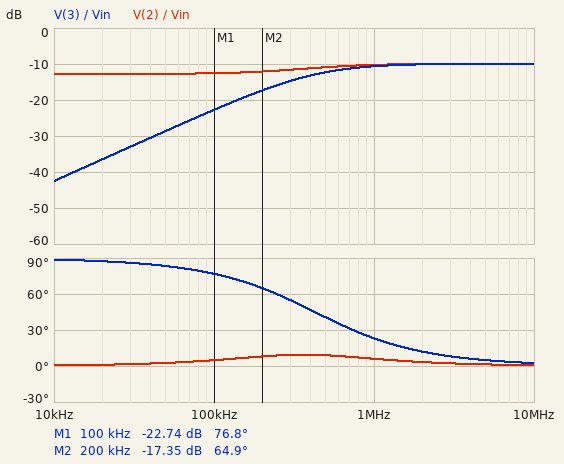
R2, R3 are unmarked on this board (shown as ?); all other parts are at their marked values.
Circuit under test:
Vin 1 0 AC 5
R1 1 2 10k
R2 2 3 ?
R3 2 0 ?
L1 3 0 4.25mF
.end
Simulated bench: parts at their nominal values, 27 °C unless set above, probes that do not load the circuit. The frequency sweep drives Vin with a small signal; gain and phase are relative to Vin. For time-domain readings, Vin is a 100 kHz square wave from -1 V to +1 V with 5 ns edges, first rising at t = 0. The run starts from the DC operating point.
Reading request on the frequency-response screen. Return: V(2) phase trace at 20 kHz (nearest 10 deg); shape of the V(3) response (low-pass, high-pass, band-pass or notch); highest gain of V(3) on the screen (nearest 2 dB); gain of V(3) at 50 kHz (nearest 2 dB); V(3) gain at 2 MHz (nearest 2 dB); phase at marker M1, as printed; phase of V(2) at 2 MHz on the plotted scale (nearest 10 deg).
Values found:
0 deg
high-pass
-10 dB
-28 dB
-10 dB
76.8 deg
0 deg
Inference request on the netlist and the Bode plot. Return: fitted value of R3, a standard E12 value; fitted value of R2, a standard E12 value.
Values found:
4.7 kΩ
8.2 kΩ
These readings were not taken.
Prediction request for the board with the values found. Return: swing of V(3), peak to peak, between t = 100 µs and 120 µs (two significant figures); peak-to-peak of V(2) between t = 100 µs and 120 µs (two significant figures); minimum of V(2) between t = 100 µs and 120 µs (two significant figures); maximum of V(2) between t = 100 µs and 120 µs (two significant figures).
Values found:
1.3 V
820 mV
-410 mV
410 mV
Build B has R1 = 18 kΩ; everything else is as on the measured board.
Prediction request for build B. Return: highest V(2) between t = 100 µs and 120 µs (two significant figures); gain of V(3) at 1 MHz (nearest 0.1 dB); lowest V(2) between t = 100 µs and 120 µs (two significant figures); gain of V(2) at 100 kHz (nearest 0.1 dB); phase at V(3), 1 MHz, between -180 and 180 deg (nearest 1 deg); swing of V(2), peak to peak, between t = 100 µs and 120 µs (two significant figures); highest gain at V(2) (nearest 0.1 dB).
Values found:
270 mV
-14.5 dB
-270 mV
-16.7 dB
24 deg
540 mV
-13.7 dB
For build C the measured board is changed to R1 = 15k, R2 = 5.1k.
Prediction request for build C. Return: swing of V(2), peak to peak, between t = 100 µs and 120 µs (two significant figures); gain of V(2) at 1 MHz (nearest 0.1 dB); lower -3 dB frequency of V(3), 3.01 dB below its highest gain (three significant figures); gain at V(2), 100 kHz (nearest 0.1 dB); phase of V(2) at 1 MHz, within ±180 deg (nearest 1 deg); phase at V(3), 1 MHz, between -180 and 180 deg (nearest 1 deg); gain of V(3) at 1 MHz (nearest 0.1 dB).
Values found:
670 mV
-12.7 dB
325 kHz
-16.4 dB
7 deg
18 deg
-12.9 dB
